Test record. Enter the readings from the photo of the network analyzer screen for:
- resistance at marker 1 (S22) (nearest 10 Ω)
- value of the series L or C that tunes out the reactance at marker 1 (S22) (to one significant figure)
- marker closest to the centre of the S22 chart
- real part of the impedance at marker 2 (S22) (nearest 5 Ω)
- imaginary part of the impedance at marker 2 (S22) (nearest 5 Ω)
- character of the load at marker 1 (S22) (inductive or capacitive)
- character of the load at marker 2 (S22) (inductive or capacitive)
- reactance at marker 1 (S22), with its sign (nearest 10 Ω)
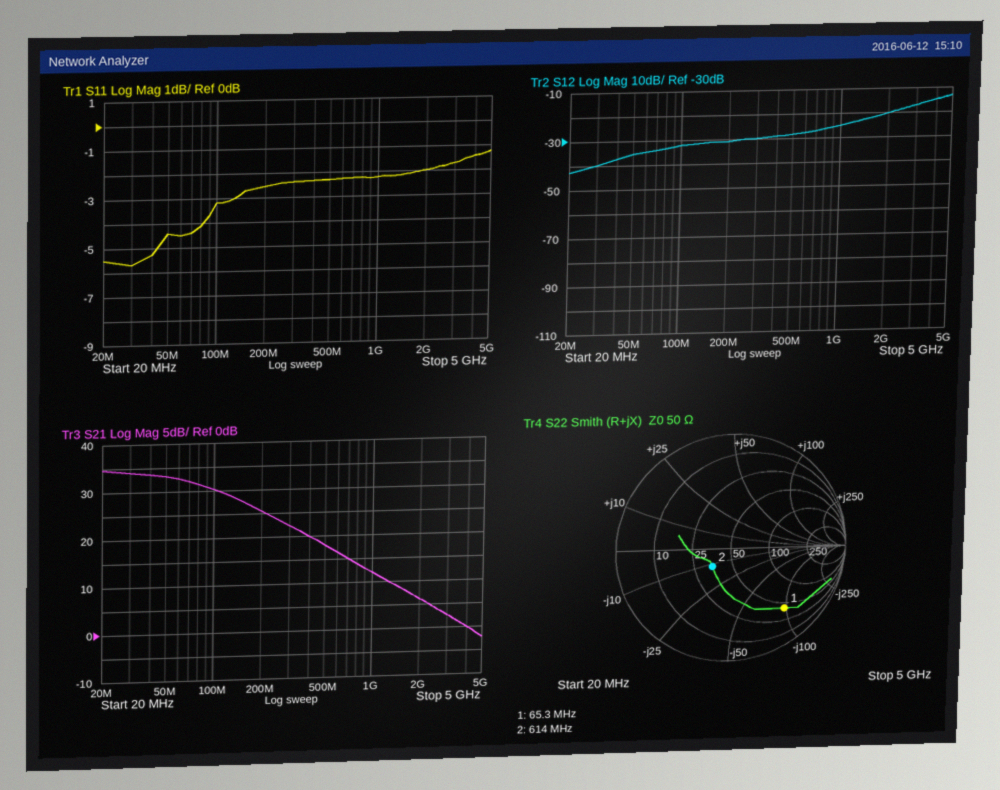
40 Ω
200 nH
marker 2
35 Ω
-10 Ω
capacitive
capacitive
-100 Ω
